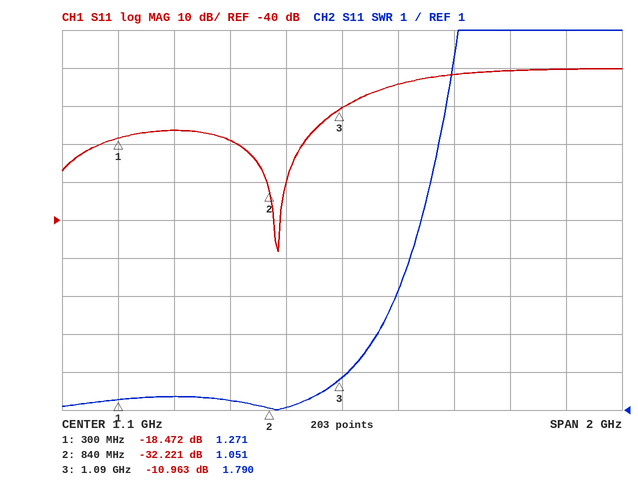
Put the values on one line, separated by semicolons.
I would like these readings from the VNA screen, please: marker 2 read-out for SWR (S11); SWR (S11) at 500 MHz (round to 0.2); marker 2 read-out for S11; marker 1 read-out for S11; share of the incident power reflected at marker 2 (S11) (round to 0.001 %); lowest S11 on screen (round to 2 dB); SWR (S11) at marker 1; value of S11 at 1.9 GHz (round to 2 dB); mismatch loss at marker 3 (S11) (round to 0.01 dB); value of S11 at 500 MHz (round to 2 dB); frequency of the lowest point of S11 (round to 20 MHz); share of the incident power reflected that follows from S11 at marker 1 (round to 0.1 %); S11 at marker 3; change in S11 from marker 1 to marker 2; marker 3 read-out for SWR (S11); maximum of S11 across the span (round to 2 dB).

1.051; 1.4; -32.221 dB; -18.472 dB; 0.060 %; -48 dB; 1.271; 0 dB; 0.36 dB; -16 dB; 880 MHz; 1.4 %; -10.963 dB; -13.749 dB; 1.790; 0 dB
